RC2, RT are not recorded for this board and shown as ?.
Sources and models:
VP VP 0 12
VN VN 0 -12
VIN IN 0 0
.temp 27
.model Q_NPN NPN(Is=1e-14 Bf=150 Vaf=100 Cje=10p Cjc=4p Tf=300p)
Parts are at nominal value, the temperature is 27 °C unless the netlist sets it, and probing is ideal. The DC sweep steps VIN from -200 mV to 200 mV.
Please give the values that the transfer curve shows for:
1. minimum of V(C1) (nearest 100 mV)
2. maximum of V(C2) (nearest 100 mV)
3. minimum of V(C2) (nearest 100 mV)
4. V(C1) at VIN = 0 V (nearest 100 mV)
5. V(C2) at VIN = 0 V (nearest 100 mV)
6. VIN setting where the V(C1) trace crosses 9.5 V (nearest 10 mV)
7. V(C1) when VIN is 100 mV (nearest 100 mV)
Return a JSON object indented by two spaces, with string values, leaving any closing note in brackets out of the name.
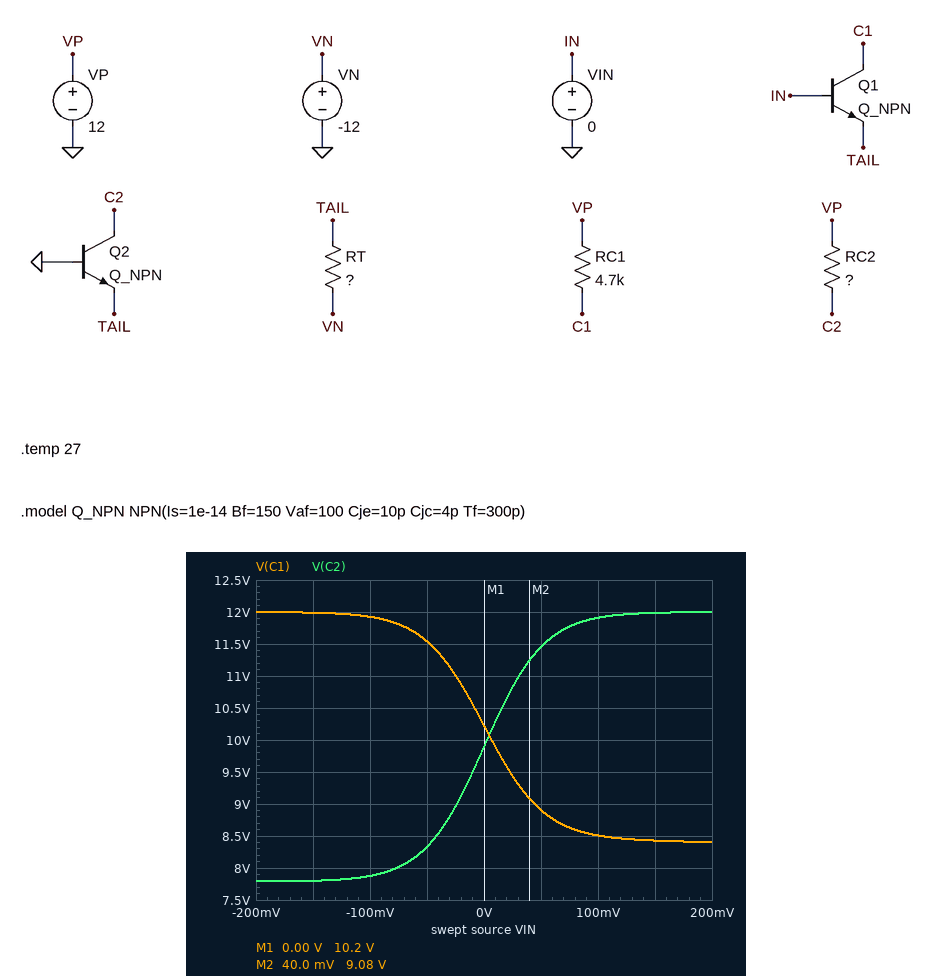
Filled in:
{
  "minimum of V(C1)": "8.4 V",
  "maximum of V(C2)": "12.0 V",
  "minimum of V(C2)": "7.8 V",
  "V(C1) at VIN = 0 V": "10.2 V",
  "V(C2) at VIN = 0 V": "9.9 V",
  "VIN setting where the V(C1) trace crosses 9.5 V": "20 mV",
  "V(C1) when VIN is 100 mV": "8.5 V"
}
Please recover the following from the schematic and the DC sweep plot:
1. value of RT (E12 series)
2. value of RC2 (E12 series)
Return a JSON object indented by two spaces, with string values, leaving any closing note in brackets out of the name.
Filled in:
{
  "value of RT": "15 kΩ",
  "value of RC2": "5.6 kΩ"
}
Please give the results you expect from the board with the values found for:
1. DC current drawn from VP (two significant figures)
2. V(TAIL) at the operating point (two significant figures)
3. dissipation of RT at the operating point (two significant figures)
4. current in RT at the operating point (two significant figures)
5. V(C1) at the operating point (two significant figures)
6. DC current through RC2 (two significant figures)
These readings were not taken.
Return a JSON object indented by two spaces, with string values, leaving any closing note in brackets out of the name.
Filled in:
{
  "DC current drawn from VP": "750 µA",
  "V(TAIL) at the operating point": "-630 mV",
  "dissipation of RT at the operating point": "8.6 mW",
  "current in RT at the operating point": "760 µA",
  "V(C1) at the operating point": "10 V",
  "DC current through RC2": "380 µA"
}
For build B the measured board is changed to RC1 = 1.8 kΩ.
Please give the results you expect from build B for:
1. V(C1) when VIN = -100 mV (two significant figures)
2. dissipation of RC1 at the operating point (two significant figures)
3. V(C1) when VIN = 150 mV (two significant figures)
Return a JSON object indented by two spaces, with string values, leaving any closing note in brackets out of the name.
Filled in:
{
  "V(C1) when VIN = -100 mV": "12 V",
  "dissipation of RC1 at the operating point": "260 µW",
  "V(C1) when VIN = 150 mV": "11 V"
}
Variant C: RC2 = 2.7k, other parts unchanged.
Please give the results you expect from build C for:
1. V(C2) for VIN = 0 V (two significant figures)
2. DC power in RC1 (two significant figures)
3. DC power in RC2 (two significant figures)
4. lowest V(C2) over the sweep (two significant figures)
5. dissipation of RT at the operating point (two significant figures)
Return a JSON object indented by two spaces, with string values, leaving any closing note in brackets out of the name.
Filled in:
{
  "V(C2) for VIN = 0 V": "11 V",
  "DC power in RC1": "660 µW",
  "DC power in RC2": "390 µW",
  "lowest V(C2) over the sweep": "10 V",
  "dissipation of RT at the operating point": "8.6 mW"
}
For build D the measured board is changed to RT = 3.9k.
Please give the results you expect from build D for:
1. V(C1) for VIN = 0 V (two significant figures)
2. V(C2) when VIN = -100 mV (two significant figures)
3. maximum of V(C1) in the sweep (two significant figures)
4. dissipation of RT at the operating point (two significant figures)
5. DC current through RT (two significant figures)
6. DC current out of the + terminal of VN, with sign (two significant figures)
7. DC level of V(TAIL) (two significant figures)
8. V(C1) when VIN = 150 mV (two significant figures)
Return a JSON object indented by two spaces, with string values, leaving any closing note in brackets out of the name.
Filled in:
{
  "V(C1) for VIN = 0 V": "5.2 V",
  "V(C2) when VIN = -100 mV": "-640 mV",
  "maximum of V(C1) in the sweep": "12 V",
  "dissipation of RT at the operating point": "33 mW",
  "DC current through RT": "2.9 mA",
  "DC current out of the + terminal of VN, with sign": "-2.9 mA",
  "DC level of V(TAIL)": "-660 mV",
  "V(C1) when VIN = 150 mV": "-470 mV"
}
